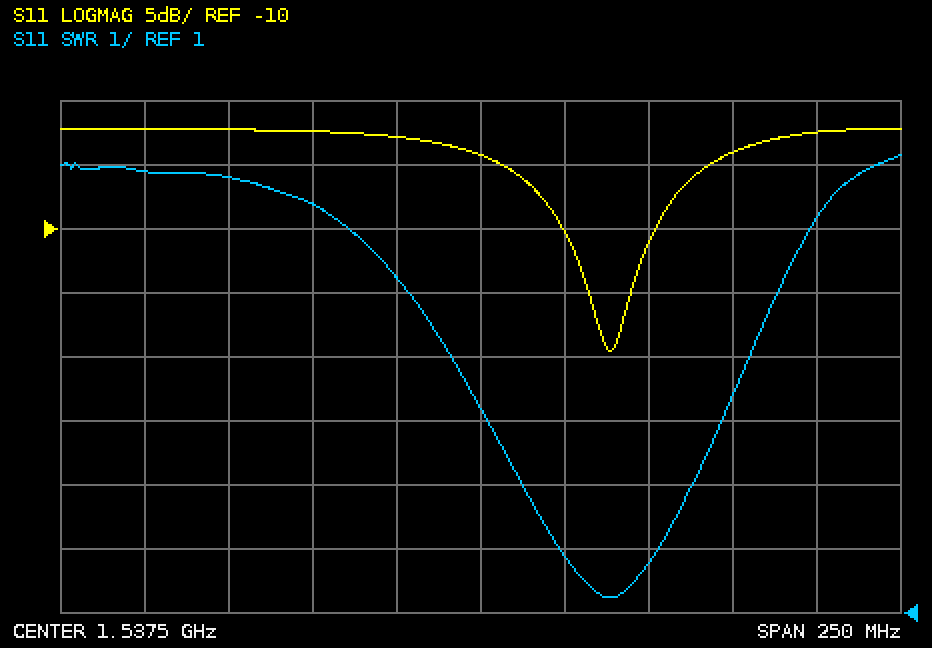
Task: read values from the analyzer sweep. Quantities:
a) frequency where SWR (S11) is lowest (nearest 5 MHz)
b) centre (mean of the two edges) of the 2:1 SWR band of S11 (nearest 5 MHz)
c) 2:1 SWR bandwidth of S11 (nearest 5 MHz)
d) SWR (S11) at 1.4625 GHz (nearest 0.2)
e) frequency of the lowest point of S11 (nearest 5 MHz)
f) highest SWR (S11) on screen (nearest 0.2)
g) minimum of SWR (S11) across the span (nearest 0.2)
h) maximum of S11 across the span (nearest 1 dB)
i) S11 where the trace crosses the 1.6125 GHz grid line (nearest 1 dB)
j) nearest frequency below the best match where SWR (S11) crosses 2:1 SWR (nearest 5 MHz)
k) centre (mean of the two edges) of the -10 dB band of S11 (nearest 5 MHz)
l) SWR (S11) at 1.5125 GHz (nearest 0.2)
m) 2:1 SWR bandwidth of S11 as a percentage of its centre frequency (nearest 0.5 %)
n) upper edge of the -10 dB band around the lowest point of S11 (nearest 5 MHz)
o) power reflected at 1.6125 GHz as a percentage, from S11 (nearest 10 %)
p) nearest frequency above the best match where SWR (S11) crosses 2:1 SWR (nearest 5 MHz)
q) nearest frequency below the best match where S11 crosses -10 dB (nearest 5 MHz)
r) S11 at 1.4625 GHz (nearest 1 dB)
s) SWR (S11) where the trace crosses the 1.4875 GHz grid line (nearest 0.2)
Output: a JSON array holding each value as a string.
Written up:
["1.575 GHz", "1.575 GHz", "30 MHz", "7.8", "1.575 GHz", "8.2", "1.2", "-2 dB", "-4 dB", "1.560 GHz", "1.575 GHz", "6.2", "2.0 %", "1.590 GHz", "40 %", "1.590 GHz", "1.560 GHz", "-2 dB", "7.4"]
